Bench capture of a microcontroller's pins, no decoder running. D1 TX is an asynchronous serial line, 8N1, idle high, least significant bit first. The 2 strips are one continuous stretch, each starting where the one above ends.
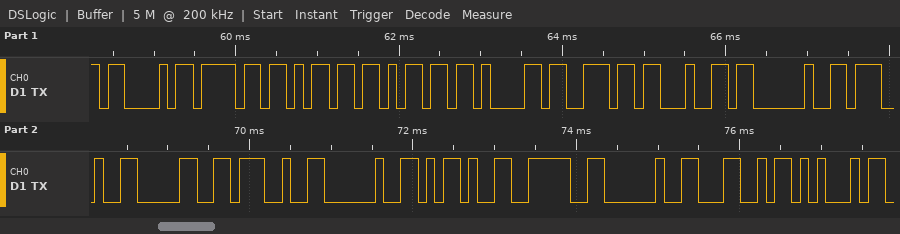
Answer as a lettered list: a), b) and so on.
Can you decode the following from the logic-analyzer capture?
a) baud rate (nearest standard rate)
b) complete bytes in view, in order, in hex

a) 9600 baud
b) 0x43 0x6F 0x6D 0x6D 0x61 0x6E 0x64 0x20 0x27 0x30 0x27 0x20 0x2D 0x3E 0x20 0x4C 0x45
